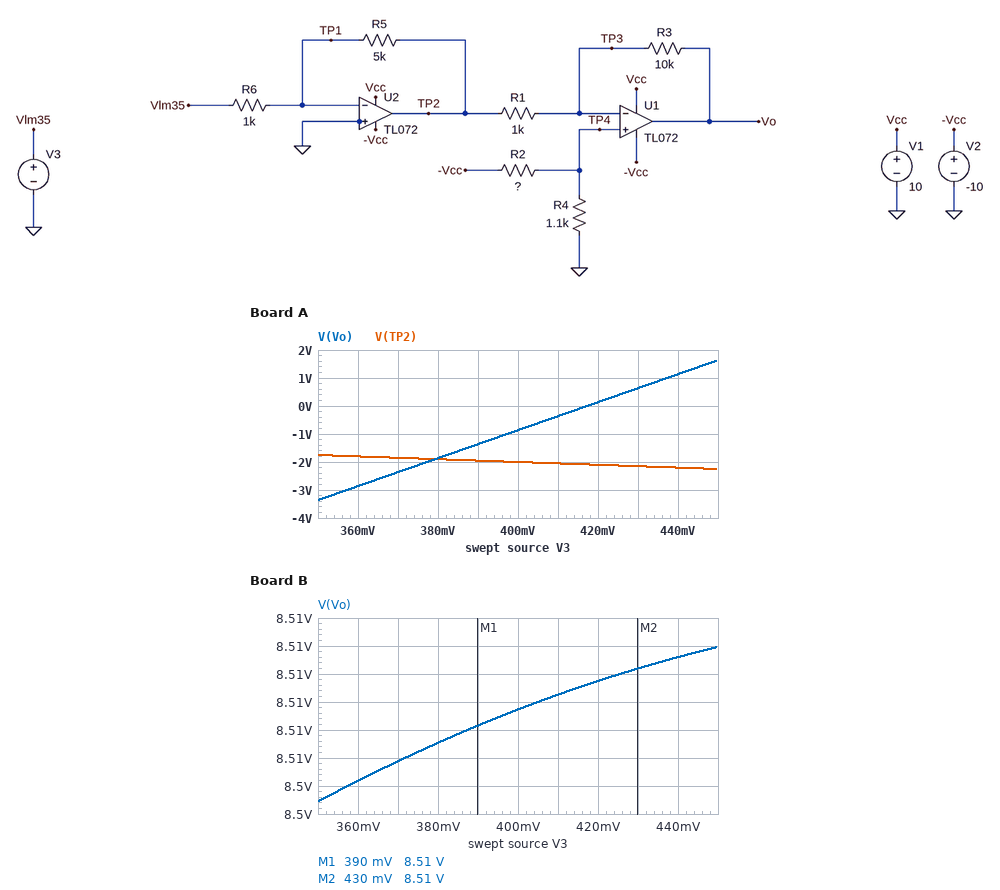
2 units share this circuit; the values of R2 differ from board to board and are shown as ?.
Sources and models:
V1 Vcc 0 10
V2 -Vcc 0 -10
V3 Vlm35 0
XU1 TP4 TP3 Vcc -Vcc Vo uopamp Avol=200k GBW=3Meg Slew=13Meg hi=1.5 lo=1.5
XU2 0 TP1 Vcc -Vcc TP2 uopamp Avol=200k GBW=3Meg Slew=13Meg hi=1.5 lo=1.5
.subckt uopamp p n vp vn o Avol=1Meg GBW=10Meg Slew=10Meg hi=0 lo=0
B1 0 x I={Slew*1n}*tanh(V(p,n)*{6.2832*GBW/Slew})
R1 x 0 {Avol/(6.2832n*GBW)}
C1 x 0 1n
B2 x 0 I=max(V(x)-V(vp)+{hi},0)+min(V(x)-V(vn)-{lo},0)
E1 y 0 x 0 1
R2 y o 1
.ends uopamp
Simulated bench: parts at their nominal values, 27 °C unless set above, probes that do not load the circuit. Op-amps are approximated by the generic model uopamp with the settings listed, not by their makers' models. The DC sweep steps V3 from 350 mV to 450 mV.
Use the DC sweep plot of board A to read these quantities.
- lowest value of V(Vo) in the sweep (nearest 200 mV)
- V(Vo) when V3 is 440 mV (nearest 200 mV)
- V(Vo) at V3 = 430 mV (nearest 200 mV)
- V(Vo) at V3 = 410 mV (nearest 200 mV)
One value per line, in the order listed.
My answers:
-3.4 V
1.2 V
600 mV
-400 mV
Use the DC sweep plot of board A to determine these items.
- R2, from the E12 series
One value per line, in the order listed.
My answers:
4.7 kΩ
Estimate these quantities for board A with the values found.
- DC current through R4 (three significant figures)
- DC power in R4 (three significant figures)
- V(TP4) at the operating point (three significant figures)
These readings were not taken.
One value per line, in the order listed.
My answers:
1.72 mA
3.27 mW
-1.90 V
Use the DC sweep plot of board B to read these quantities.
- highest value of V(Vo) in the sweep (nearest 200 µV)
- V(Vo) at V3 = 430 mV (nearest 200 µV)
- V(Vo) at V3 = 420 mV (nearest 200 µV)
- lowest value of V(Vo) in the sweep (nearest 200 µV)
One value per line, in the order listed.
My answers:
8.5090 V
8.5082 V
8.5078 V
8.5034 V
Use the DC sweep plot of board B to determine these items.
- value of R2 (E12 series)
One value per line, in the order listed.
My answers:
18 kΩ
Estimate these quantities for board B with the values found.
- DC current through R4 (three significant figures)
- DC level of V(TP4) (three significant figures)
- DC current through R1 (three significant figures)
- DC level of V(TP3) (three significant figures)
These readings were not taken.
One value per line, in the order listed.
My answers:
524 µA
-576 mV
576 µA
-576 mV
